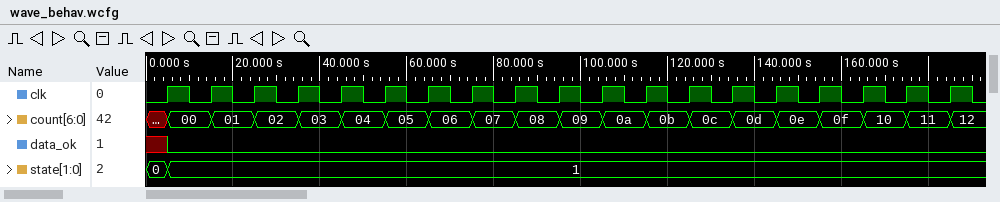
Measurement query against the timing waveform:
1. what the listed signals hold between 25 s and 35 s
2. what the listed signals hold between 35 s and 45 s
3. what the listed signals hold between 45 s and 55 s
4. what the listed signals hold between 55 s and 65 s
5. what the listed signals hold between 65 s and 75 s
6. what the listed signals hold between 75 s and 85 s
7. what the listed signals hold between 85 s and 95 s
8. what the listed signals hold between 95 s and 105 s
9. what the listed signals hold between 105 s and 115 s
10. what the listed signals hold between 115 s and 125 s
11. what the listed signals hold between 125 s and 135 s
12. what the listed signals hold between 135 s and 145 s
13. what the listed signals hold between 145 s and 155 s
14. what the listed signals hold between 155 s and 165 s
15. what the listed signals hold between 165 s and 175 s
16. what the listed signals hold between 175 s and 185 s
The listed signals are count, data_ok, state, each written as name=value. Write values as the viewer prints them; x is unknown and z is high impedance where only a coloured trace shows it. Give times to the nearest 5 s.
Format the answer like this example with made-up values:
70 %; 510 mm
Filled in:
count=02, data_ok=0, state=1; count=03, data_ok=0, state=1; count=04, data_ok=0, state=1; count=05, data_ok=0, state=1; count=06, data_ok=0, state=1; count=07, data_ok=0, state=1; count=08, data_ok=0, state=1; count=09, data_ok=0, state=1; count=0a, data_ok=0, state=1; count=0b, data_ok=0, state=1; count=0c, data_ok=0, state=1; count=0d, data_ok=0, state=1; count=0e, data_ok=0, state=1; count=0f, data_ok=0, state=1; count=10, data_ok=0, state=1; count=11, data_ok=0, state=1
